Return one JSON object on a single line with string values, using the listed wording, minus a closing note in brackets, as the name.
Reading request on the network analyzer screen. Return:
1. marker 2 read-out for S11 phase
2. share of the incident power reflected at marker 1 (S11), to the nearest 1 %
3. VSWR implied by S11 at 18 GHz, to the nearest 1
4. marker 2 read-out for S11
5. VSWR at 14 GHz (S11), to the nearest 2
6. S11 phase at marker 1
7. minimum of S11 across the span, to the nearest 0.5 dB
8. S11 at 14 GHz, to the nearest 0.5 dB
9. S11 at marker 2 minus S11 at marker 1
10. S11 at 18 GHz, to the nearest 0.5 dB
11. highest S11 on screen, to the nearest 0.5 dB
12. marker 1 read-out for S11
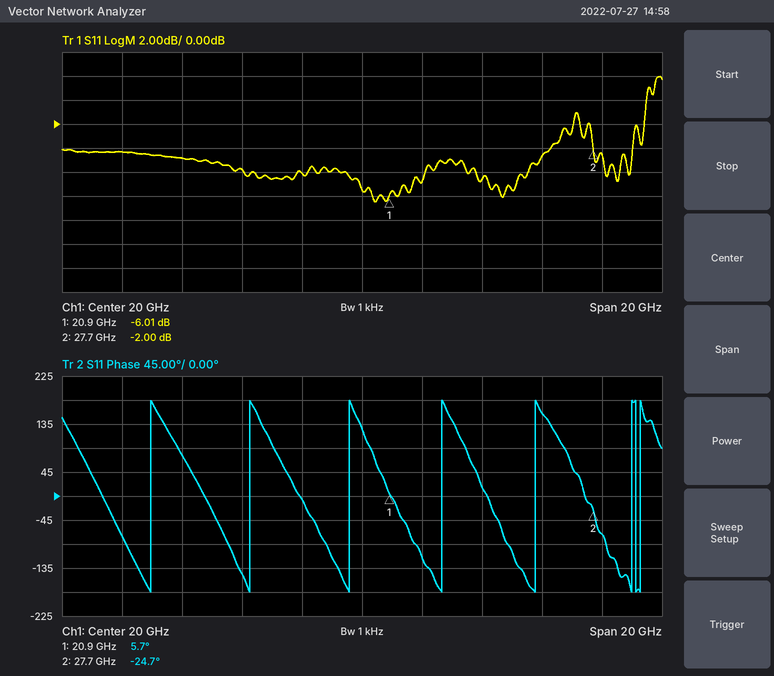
{"marker 2 read-out for S11 phase": "-24.7°", "share of the incident power reflected at marker 1 (S11), to the nearest 1 %": "25 %", "VSWR implied by S11 at 18 GHz, to the nearest 1": "4", "marker 2 read-out for S11": "-2.00 dB", "VSWR at 14 GHz (S11), to the nearest 2": "6", "S11 phase at marker 1": "5.7°", "minimum of S11 across the span, to the nearest 0.5 dB": "-6.5 dB", "S11 at 14 GHz, to the nearest 0.5 dB": "-3.0 dB", "S11 at marker 2 minus S11 at marker 1": "4.01 dB", "S11 at 18 GHz, to the nearest 0.5 dB": "-4.0 dB", "highest S11 on screen, to the nearest 0.5 dB": "4.0 dB", "marker 1 read-out for S11": "-6.01 dB"}
